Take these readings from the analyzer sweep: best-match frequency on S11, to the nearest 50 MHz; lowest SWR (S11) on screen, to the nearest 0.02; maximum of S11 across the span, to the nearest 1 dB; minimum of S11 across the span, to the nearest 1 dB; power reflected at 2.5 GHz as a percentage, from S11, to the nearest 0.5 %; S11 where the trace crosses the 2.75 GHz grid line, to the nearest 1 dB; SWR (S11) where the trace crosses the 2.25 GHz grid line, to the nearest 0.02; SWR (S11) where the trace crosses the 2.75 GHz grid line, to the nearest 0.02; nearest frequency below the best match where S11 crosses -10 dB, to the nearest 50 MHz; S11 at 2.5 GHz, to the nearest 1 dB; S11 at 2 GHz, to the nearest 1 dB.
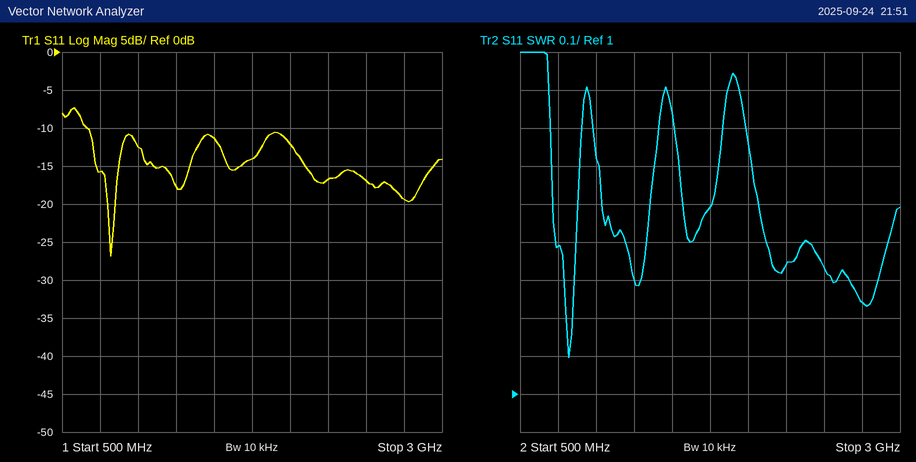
800 MHz
1.10
-7 dB
-27 dB
2.0 %
-19 dB
1.34
1.24
650 MHz
-17 dB
-12 dB
